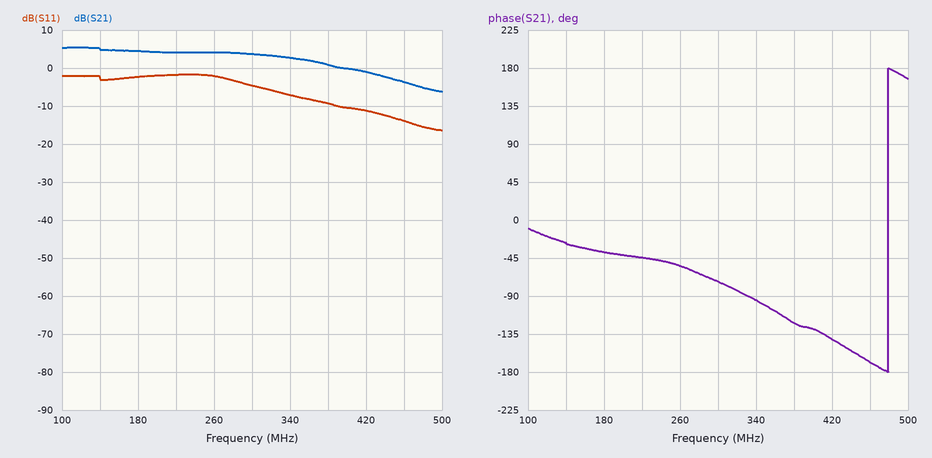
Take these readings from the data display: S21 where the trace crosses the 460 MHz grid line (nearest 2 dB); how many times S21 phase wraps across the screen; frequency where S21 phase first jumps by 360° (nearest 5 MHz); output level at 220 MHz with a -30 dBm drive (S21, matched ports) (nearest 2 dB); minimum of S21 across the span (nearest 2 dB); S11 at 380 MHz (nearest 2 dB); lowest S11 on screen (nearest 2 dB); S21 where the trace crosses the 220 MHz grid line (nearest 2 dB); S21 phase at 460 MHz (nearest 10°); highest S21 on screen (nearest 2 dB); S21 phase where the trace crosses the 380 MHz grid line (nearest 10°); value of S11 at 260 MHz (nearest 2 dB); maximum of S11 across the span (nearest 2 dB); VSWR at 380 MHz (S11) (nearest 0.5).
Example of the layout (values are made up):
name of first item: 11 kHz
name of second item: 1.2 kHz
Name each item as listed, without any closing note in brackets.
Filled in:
S21 where the trace crosses the 460 MHz grid line: -4 dB
how many times S21 phase wraps across the screen: 1
frequency where S21 phase first jumps by 360°: 480 MHz
output level at 220 MHz with a -30 dBm drive (S21, matched ports): -26 dBm
minimum of S21 across the span: -6 dB
S11 at 380 MHz: -10 dB
lowest S11 on screen: -16 dB
S21 where the trace crosses the 220 MHz grid line: 4 dB
S21 phase at 460 MHz: -170°
highest S21 on screen: 6 dB
S21 phase where the trace crosses the 380 MHz grid line: -120°
value of S11 at 260 MHz: -2 dB
maximum of S11 across the span: -2 dB
VSWR at 380 MHz (S11): 2.0
